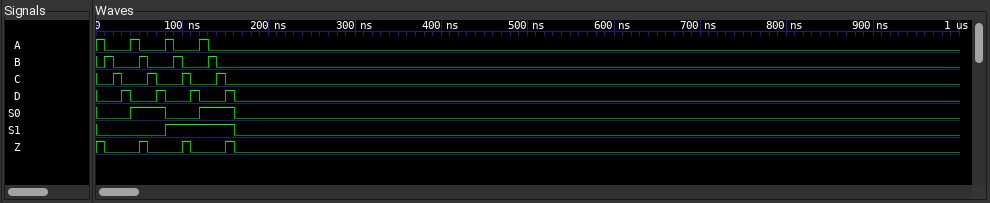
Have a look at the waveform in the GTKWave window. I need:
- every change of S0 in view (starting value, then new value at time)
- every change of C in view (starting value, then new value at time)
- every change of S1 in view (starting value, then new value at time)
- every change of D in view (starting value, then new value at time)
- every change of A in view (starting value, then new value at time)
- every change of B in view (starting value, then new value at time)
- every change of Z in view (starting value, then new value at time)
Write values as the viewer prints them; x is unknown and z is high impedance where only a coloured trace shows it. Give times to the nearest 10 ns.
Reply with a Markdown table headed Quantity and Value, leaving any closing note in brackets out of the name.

| Quantity | Value |
|---|---|
| every change of S0 in view | 0, 1 at 40 ns, 0 at 80 ns, 1 at 120 ns, 0 at 160 ns |
| every change of C in view | 0, 1 at 20 ns, 0 at 30 ns, 1 at 60 ns, 0 at 70 ns, 1 at 100 ns, 0 at 110 ns, 1 at 140 ns, 0 at 150 ns |
| every change of S1 in view | 0, 1 at 80 ns, 0 at 160 ns |
| every change of D in view | 0, 1 at 30 ns, 0 at 40 ns, 1 at 70 ns, 0 at 80 ns, 1 at 110 ns, 0 at 120 ns, 1 at 150 ns, 0 at 160 ns |
| every change of A in view | 1, 0 at 10 ns, 1 at 40 ns, 0 at 50 ns, 1 at 80 ns, 0 at 90 ns, 1 at 120 ns, 0 at 130 ns |
| every change of B in view | 0, 1 at 10 ns, 0 at 20 ns, 1 at 50 ns, 0 at 60 ns, 1 at 90 ns, 0 at 100 ns, 1 at 130 ns, 0 at 140 ns |
| every change of Z in view | 1, 0 at 10 ns, 1 at 50 ns, 0 at 60 ns, 1 at 100 ns, 0 at 110 ns, 1 at 150 ns, 0 at 160 ns |
